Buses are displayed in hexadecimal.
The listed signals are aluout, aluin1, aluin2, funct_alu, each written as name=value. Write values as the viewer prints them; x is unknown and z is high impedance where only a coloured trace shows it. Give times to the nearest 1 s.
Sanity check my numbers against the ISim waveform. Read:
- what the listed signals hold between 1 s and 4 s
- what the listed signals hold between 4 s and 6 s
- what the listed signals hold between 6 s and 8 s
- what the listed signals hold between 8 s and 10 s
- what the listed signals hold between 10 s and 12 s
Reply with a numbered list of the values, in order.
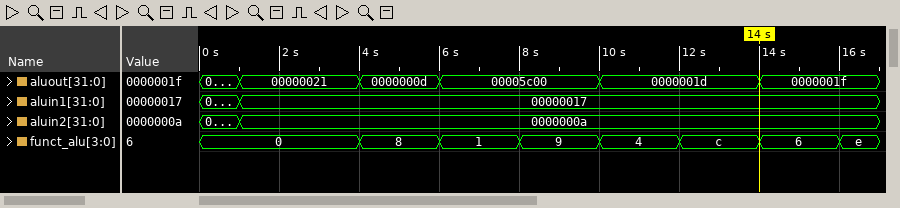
1. aluout=00000021, aluin1=00000017, aluin2=0000000a, funct_alu=0
2. aluout=0000000d, aluin1=00000017, aluin2=0000000a, funct_alu=8
3. aluout=00005c00, aluin1=00000017, aluin2=0000000a, funct_alu=1
4. aluout=00005c00, aluin1=00000017, aluin2=0000000a, funct_alu=9
5. aluout=0000001d, aluin1=00000017, aluin2=0000000a, funct_alu=4
